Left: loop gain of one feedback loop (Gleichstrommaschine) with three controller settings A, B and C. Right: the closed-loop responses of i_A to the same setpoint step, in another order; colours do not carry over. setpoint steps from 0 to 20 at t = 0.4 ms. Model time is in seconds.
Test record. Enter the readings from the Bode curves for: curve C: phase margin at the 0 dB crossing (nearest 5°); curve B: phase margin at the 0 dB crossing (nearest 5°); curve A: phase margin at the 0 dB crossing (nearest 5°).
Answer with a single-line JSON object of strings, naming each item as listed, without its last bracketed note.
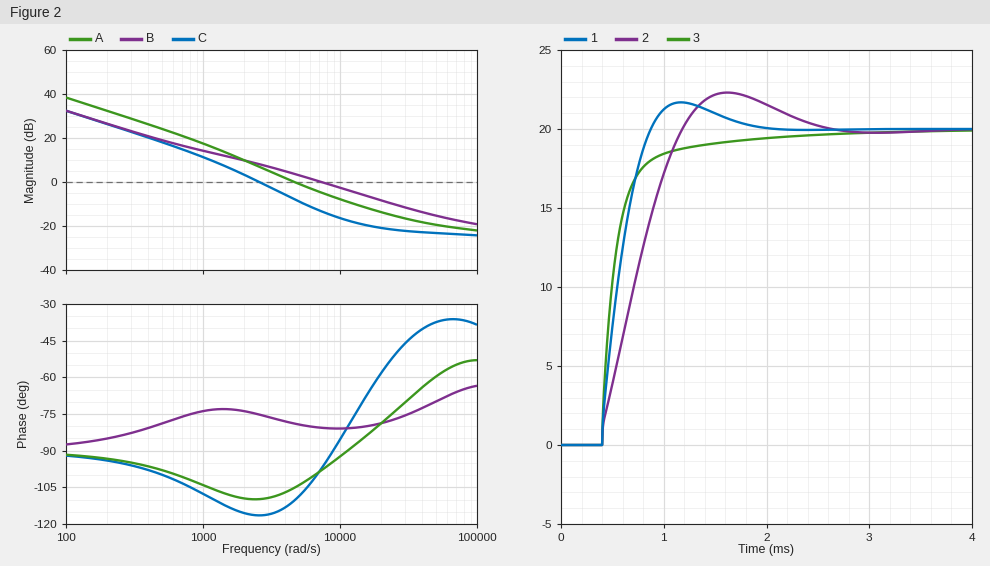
{"curve C: phase margin at the 0 dB crossing": "65°", "curve B: phase margin at the 0 dB crossing": "100°", "curve A: phase margin at the 0 dB crossing": "75°"}
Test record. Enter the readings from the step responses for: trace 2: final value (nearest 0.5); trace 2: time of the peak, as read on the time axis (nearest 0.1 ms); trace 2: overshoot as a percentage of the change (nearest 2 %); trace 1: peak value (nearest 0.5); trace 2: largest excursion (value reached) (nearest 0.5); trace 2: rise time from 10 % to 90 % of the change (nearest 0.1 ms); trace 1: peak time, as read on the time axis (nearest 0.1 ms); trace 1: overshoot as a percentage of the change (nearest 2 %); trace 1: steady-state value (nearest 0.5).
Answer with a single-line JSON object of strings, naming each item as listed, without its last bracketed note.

{"trace 2: final value": "20.0", "trace 2: time of the peak, as read on the time axis": "1.6 ms", "trace 2: overshoot as a percentage of the change": "12 %", "trace 1: peak value": "21.5", "trace 2: largest excursion (value reached)": "22.5", "trace 2: rise time from 10 % to 90 % of the change": "0.6 ms", "trace 1: peak time, as read on the time axis": "1.2 ms", "trace 1: overshoot as a percentage of the change": "8 %", "trace 1: steady-state value": "20.0"}
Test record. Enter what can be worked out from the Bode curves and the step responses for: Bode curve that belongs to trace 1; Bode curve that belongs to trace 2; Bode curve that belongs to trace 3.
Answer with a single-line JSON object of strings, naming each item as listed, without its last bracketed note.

{"Bode curve that belongs to trace 1": "A", "Bode curve that belongs to trace 2": "C", "Bode curve that belongs to trace 3": "B"}
